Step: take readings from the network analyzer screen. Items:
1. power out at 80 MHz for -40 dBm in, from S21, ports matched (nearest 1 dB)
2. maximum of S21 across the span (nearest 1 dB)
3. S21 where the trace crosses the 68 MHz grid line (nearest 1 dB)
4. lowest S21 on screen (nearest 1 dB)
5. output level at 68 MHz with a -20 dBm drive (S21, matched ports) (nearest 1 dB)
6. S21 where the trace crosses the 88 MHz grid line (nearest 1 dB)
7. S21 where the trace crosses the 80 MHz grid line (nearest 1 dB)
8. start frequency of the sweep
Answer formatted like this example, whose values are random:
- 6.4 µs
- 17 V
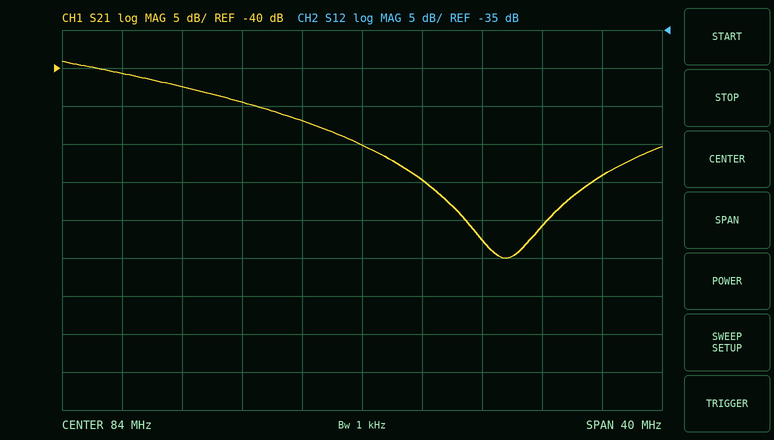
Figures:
- -87 dBm
- -39 dB
- -41 dB
- -65 dB
- -61 dBm
- -55 dB
- -47 dB
- 64 MHz
